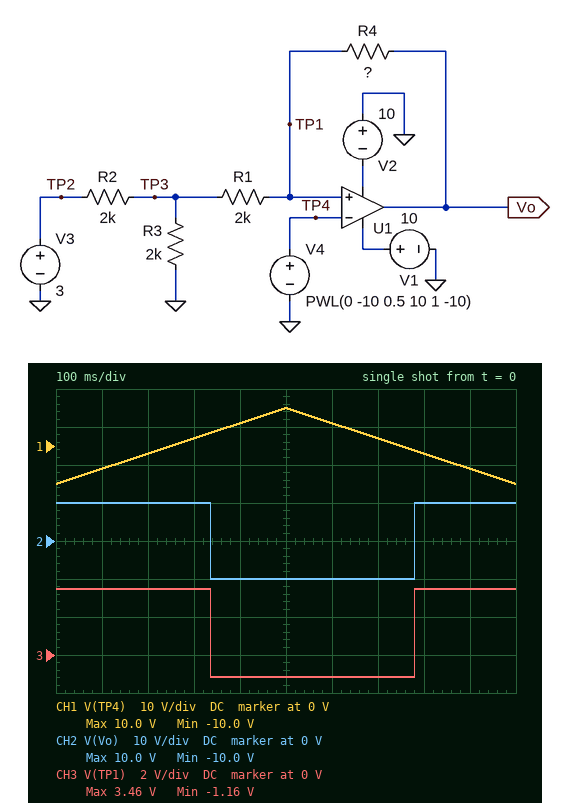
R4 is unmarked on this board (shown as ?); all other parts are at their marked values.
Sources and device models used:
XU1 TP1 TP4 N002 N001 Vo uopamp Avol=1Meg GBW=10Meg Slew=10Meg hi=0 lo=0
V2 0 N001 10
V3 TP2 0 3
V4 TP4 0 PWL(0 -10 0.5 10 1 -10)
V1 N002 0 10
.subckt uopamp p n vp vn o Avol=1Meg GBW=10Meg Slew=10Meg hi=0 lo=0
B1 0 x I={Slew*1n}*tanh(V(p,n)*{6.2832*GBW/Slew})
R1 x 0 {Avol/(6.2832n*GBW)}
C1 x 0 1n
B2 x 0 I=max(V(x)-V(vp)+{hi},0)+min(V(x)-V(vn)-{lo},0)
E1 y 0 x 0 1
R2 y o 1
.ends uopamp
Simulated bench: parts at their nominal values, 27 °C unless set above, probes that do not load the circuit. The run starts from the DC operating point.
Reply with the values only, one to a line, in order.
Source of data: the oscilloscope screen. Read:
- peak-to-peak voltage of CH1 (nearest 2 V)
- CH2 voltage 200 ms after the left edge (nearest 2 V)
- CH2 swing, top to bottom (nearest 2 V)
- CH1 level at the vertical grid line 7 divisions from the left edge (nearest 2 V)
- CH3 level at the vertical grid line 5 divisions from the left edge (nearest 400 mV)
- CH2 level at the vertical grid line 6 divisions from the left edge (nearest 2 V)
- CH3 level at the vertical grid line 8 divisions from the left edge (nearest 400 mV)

20 V
10 V
20 V
2 V
-1.2 V
-10 V
3.6 V
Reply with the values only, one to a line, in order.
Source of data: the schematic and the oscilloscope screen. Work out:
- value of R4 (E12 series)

10 kΩ
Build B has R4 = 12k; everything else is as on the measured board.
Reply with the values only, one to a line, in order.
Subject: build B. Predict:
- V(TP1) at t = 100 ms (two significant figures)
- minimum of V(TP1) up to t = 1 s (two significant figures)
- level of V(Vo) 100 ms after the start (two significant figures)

3.2 V
-800 mV
10 V
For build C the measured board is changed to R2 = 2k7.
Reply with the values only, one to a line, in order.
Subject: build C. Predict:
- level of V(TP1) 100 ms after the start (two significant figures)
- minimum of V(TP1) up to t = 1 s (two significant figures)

3.4 V
-1.4 V
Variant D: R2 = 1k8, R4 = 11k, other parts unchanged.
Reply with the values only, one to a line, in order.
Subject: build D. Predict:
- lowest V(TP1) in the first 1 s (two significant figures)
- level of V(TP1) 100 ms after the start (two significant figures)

-870 mV
3.4 V
